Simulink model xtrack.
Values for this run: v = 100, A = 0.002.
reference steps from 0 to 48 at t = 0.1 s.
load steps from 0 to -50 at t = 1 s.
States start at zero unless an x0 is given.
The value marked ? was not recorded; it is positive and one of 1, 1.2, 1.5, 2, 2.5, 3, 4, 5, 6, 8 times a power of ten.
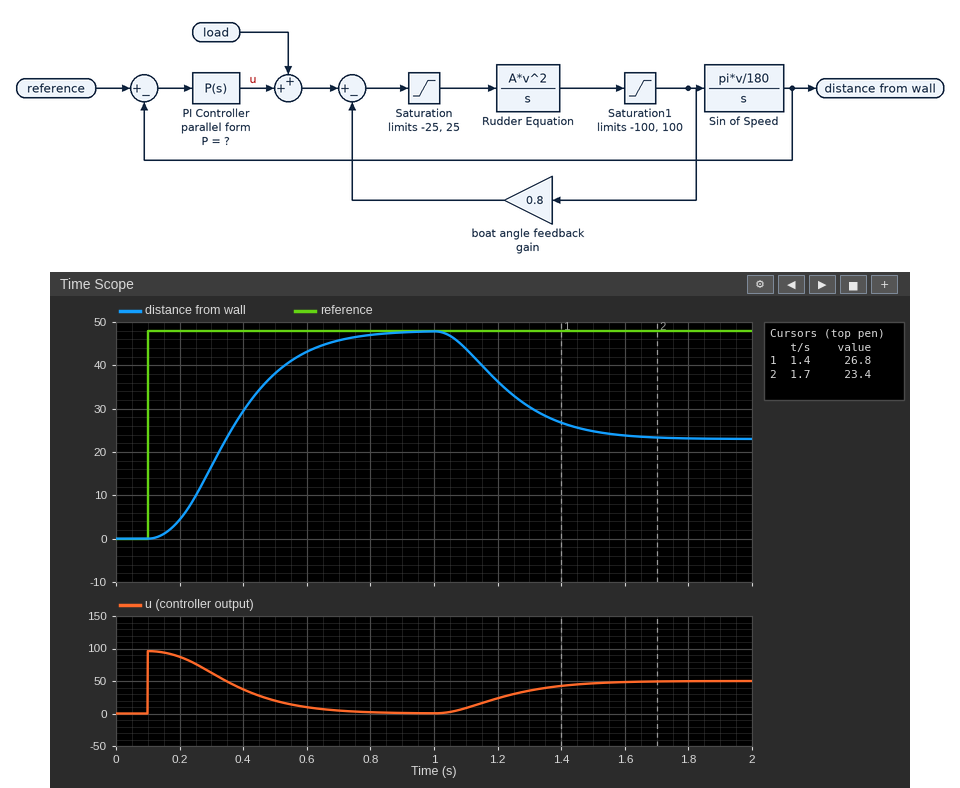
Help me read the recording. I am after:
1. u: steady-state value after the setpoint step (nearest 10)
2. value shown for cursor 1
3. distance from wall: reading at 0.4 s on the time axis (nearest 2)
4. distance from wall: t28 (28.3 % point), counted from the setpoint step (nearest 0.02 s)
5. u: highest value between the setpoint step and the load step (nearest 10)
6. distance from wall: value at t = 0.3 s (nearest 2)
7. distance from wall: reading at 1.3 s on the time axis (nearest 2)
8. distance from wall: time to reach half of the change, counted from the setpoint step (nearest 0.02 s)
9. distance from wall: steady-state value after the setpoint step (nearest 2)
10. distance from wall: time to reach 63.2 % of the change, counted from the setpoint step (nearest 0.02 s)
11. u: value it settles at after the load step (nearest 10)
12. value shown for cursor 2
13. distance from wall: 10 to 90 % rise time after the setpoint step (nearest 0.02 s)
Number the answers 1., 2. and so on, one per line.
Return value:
1. 0
2. 26.8
3. 30
4. 0.18 s
5. 100
6. 16
7. 30
8. 0.26 s
9. 48
10. 0.30 s
11. 50
12. 23.4
13. 0.40 s
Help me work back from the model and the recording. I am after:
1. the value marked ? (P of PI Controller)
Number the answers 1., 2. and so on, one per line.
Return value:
1. 2
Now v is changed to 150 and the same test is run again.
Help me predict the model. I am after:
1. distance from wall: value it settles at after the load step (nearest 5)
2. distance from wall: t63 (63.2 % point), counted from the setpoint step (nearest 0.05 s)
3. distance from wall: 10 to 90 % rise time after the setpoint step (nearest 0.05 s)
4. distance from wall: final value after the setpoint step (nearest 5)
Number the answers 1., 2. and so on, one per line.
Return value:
1. 25
2. 0.20 s
3. 0.30 s
4. 50
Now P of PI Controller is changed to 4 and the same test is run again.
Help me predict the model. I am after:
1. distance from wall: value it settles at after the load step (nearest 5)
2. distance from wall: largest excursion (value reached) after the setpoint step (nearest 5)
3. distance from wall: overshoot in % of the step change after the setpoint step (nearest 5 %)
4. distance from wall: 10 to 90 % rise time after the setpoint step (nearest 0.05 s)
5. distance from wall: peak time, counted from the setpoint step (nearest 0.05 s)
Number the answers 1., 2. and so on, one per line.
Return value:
1. 35
2. 55
3. 15 %
4. 0.25 s
5. 0.50 s
